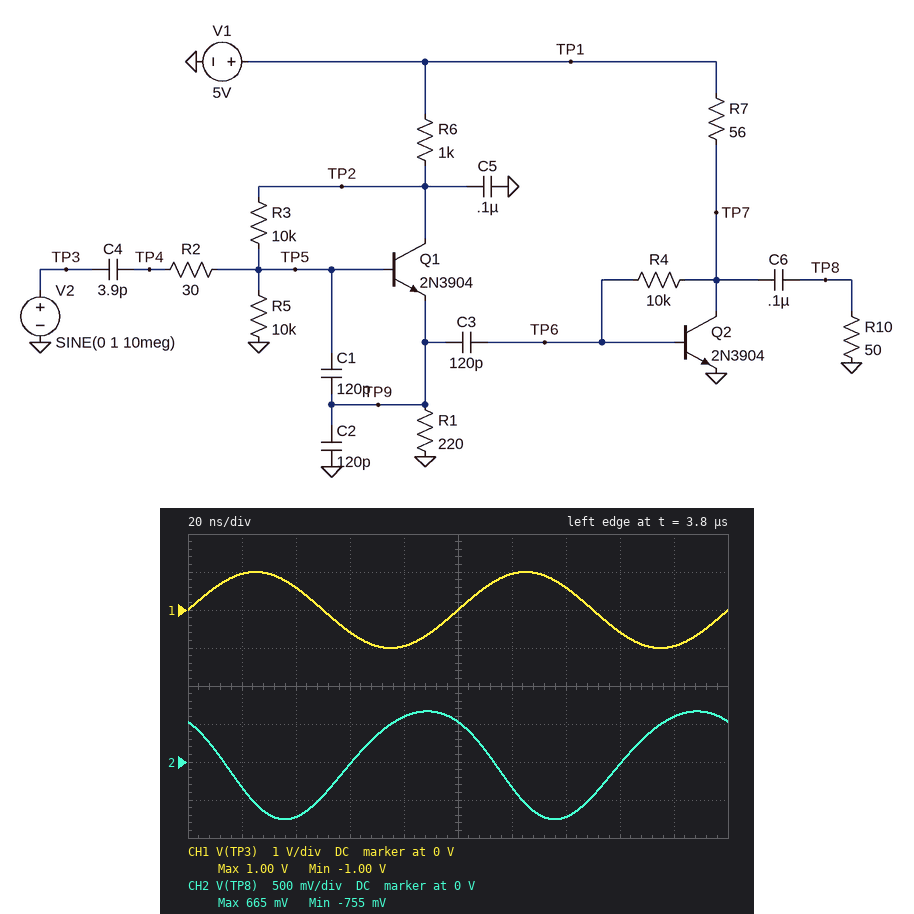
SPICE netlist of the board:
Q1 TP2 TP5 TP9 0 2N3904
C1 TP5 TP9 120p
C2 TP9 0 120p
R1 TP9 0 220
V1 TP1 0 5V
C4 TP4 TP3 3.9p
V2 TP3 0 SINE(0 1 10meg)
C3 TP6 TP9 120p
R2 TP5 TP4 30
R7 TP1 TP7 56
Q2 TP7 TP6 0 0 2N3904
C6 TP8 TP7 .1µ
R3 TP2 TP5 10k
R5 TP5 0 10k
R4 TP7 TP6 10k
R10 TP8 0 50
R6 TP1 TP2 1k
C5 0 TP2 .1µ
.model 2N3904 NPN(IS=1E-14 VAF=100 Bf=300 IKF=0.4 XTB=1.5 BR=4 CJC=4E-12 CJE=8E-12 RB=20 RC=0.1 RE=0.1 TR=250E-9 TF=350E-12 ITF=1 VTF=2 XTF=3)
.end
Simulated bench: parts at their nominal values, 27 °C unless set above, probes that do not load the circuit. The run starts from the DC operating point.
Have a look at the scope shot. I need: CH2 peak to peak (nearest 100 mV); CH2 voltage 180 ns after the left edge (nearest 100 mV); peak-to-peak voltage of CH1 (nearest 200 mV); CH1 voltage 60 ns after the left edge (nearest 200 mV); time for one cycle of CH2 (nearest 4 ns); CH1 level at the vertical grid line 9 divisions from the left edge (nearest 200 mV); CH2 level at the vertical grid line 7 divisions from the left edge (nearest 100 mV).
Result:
1.4 V
600 mV
2.0 V
-600 mV
100 ns
-1.0 V
-700 mV
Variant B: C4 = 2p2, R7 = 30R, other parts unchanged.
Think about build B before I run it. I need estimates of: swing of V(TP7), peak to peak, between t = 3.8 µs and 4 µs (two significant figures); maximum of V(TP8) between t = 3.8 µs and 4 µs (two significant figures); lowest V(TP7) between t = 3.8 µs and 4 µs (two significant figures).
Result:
680 mV
330 mV
2.8 V
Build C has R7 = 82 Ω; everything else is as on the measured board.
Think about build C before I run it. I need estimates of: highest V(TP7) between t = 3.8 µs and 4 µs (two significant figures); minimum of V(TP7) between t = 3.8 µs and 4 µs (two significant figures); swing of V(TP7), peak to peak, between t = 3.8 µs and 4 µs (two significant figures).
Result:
2.8 V
1.2 V
1.6 V
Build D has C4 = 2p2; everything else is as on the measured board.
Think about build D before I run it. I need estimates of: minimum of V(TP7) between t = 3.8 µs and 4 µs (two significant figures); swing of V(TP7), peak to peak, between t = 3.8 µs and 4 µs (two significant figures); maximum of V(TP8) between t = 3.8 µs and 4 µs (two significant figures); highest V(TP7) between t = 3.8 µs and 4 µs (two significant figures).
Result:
2.0 V
880 mV
430 mV
2.9 V
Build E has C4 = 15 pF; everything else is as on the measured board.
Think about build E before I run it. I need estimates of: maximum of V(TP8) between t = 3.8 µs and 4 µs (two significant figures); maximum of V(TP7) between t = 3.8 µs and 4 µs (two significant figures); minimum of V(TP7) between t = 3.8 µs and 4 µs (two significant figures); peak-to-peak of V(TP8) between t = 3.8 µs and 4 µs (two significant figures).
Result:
1.1 V
3.6 V
780 mV
2.8 V
